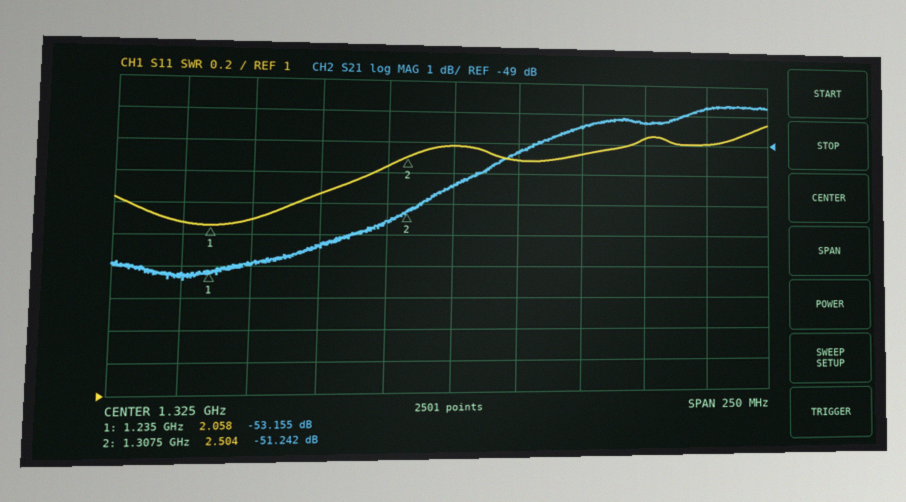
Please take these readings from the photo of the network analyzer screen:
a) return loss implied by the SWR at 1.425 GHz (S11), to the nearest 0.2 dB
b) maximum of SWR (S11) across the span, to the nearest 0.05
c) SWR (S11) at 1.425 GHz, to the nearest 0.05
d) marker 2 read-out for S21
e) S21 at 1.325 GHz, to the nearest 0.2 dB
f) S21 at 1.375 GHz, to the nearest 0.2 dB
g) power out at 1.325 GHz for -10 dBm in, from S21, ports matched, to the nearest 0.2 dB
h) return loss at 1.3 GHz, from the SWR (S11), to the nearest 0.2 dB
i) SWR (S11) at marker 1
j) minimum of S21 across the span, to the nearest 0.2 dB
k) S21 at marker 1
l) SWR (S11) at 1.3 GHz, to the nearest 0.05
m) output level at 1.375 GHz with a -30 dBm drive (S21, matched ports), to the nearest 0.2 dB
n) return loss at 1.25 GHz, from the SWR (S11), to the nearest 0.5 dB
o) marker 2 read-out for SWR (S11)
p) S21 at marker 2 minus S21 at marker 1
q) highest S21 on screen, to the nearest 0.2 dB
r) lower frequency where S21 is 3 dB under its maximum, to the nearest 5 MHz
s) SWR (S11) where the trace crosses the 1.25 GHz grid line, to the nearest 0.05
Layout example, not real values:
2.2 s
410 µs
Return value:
7.0 dB
2.75
2.60
-51.242 dB
-50.4 dB
-48.4 dB
-60.4 dBm
7.6 dB
2.058
-53.4 dB
-53.155 dB
2.45
-78.4 dBm
9.0 dB
2.504
1.913 dB
-47.6 dB
1.320 GHz
2.10
